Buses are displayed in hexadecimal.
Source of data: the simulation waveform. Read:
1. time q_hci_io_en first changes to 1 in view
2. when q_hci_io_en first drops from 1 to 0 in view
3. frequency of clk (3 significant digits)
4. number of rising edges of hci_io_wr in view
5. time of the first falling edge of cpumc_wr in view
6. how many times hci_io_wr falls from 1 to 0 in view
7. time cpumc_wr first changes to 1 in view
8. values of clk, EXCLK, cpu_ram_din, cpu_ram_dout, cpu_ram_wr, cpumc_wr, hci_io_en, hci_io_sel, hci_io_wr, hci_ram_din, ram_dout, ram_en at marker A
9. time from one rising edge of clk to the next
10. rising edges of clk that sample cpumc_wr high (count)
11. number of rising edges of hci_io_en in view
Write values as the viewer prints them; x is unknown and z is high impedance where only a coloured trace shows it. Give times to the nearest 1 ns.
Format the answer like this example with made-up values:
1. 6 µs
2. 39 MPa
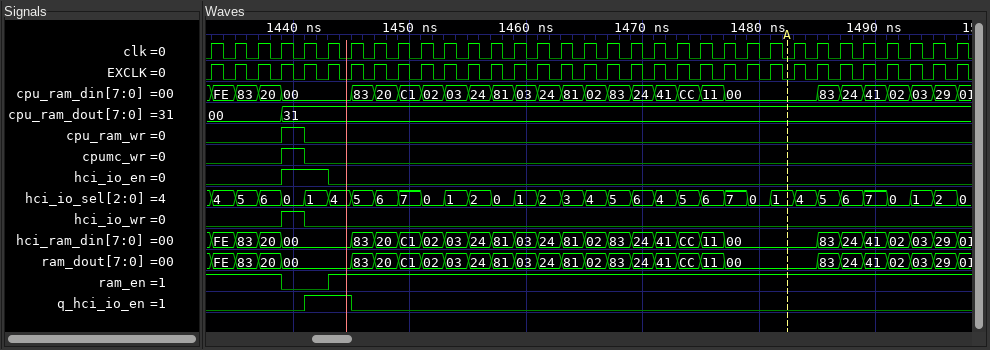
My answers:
1. 1441 ns
2. 1445 ns
3. 500 MHz
4. 1
5. 1441 ns
6. 1
7. 1439 ns
8. clk=0, EXCLK=0, cpu_ram_din=00, cpu_ram_dout=31, cpu_ram_wr=0, cpumc_wr=0, hci_io_en=0, hci_io_sel=1, hci_io_wr=0, hci_ram_din=00, ram_dout=00, ram_en=1
9. 2 ns
10. 1
11. 1
